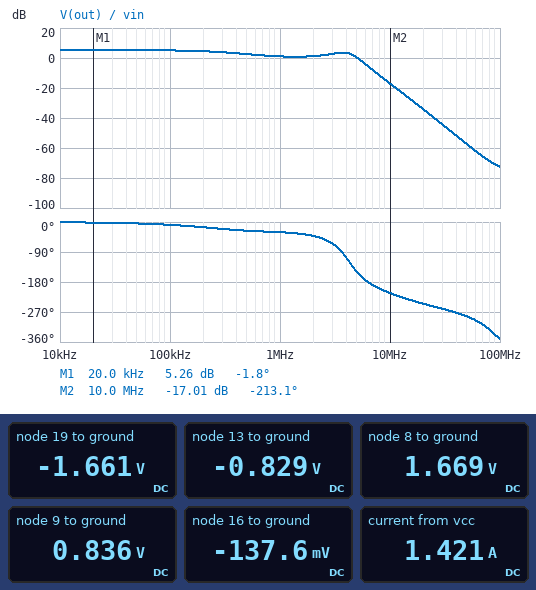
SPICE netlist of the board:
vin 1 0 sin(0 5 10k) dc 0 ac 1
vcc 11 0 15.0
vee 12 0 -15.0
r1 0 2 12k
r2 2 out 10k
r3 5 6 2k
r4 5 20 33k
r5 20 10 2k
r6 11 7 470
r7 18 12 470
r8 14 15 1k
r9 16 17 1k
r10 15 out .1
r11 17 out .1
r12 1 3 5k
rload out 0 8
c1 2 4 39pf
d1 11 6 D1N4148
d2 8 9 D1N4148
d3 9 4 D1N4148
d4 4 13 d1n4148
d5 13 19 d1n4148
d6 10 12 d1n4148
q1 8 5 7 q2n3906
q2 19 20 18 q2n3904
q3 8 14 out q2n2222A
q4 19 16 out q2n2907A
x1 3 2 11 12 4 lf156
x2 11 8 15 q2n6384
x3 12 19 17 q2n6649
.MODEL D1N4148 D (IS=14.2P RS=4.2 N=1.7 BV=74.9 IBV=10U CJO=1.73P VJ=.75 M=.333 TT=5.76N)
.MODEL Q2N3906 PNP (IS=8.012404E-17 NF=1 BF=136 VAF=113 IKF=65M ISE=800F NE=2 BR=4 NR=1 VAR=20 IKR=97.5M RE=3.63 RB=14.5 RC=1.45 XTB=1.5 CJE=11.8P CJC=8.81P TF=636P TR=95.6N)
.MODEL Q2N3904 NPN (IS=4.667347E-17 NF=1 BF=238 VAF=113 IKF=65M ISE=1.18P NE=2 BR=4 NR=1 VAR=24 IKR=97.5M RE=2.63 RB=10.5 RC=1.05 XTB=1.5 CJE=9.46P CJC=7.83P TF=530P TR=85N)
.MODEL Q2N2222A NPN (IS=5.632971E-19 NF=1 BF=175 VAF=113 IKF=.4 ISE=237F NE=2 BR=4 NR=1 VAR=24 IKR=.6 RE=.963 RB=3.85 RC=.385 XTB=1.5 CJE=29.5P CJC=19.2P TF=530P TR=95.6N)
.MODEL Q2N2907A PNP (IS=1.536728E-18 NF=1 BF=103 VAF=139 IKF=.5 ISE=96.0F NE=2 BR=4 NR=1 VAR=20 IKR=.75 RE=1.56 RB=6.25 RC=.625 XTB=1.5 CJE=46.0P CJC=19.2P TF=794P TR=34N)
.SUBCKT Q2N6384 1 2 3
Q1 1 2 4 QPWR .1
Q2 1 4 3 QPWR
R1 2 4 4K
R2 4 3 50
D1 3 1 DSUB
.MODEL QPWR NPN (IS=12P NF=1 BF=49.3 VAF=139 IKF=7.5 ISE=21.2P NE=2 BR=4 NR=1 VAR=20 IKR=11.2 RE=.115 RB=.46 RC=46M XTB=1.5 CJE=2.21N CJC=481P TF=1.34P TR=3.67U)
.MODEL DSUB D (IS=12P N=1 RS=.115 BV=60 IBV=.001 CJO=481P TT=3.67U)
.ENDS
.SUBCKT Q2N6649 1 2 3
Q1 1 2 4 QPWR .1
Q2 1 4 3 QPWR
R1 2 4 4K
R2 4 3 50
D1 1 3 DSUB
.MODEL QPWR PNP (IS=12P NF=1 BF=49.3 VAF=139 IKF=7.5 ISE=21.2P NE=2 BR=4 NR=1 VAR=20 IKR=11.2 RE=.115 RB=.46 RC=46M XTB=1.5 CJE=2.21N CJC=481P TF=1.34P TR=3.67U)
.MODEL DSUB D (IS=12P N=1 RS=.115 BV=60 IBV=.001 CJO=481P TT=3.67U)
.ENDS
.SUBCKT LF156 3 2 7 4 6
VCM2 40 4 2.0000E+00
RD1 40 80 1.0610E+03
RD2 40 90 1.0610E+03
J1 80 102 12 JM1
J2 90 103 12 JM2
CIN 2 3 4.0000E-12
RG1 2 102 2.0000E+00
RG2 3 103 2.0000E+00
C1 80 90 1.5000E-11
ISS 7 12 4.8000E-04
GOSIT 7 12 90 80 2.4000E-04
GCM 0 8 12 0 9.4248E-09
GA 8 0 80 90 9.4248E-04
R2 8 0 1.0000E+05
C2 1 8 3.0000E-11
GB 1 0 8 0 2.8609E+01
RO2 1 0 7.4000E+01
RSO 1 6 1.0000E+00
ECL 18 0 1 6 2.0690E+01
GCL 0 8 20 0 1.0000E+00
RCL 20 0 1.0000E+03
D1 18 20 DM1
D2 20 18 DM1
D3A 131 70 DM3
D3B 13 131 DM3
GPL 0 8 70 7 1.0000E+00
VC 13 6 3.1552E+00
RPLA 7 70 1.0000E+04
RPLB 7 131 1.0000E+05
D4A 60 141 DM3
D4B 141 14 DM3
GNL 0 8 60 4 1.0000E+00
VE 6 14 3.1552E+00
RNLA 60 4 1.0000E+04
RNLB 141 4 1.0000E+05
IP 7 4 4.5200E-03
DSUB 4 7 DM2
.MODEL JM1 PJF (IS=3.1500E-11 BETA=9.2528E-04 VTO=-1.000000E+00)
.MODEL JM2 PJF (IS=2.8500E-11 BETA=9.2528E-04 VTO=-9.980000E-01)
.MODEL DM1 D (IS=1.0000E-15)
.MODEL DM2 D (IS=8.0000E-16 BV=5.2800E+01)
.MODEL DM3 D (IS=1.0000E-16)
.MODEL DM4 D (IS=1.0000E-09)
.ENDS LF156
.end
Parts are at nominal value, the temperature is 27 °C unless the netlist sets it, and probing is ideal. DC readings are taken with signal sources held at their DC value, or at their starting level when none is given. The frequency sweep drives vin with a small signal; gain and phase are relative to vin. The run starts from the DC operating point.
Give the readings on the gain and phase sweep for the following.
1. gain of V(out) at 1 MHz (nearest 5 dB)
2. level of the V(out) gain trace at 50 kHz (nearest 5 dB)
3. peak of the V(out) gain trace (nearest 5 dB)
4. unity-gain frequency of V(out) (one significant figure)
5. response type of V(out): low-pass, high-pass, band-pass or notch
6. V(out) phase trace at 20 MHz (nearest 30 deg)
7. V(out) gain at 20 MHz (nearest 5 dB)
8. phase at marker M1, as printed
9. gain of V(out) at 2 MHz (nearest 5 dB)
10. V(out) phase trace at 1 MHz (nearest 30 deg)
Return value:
0 dB
5 dB
5 dB
5 MHz
low-pass
-240 deg
-35 dB
-1.8 deg
0 dB
-30 deg
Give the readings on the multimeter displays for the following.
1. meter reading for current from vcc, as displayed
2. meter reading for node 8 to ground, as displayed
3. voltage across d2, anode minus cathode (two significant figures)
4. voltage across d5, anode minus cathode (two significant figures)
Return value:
1.421 A
1.669 V
830 mV
830 mV
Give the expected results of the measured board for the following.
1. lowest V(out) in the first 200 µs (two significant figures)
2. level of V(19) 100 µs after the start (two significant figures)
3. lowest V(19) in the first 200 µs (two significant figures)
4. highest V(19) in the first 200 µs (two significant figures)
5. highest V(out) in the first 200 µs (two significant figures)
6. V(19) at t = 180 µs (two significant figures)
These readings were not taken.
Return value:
-9.2 V
-1.8 V
-11 V
7.7 V
9.2 V
-11 V
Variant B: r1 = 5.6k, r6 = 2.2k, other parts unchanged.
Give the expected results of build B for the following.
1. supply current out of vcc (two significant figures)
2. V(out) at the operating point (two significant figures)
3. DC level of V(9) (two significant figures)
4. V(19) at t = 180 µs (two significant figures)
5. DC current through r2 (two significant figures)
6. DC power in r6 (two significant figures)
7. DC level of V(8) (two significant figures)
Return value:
660 mA
5.6 mV
850 mV
-14 V
360 nA
1.1 mW
1.4 V
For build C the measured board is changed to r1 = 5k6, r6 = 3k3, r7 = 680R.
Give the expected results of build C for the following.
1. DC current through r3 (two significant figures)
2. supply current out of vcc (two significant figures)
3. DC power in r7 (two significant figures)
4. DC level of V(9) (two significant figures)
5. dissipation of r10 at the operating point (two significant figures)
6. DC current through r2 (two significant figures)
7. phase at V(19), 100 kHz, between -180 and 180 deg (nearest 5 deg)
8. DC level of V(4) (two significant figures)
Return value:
760 µA
220 mA
3.2 mW
830 mV
4.6 mW
360 nA
-10 deg
380 mV
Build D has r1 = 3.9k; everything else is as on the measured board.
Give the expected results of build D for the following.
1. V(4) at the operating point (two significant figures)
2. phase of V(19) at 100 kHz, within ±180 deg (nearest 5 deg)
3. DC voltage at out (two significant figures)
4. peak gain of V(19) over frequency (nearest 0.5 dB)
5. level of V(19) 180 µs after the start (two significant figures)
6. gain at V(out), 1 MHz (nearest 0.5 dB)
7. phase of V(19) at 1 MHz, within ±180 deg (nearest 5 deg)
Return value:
7.4 mV
-15 deg
7.1 mV
11.0 dB
-14 V
3.0 dB
-50 deg
